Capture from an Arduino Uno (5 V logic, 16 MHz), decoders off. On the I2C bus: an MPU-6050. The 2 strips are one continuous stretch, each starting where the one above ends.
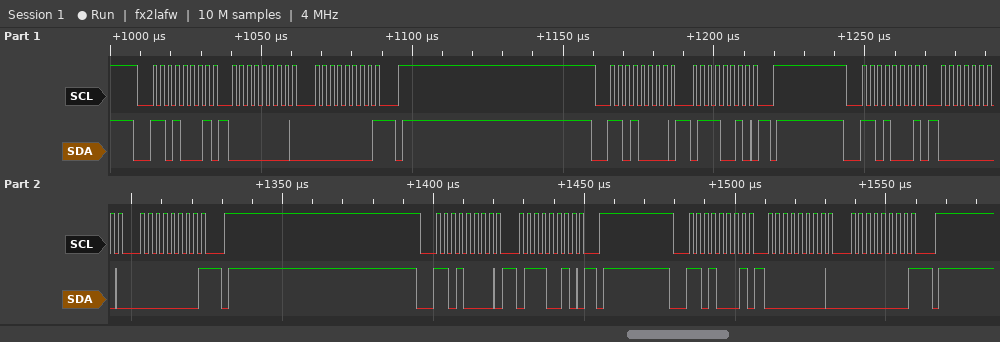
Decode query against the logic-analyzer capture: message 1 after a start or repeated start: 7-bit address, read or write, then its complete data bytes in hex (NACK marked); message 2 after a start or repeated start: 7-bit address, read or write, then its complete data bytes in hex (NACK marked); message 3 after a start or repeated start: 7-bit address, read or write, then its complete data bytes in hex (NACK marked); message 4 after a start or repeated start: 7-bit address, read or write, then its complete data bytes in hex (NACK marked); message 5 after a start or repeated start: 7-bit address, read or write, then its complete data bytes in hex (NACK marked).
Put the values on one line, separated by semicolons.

0x68 read: 00 00 NACK; 0x68 write: 72; 0x68 read: 00 00 NACK; 0x68 write: 72; 0x68 read: 00 00 NACK
